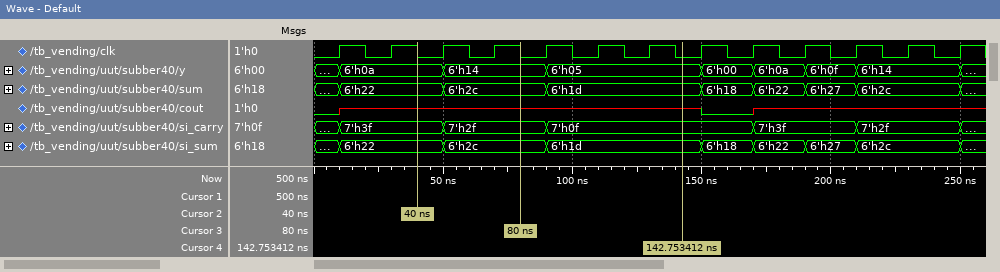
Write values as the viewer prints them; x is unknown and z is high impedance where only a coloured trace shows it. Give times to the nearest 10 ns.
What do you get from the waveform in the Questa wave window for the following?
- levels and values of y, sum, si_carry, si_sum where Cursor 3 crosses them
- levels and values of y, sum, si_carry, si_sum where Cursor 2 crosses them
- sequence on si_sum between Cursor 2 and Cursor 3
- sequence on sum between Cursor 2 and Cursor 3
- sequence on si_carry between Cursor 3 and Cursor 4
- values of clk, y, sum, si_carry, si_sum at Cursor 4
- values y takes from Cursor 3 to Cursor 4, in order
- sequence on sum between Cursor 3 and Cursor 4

y=6'h14, sum=6'h2c, si_carry=7'h2f, si_sum=6'h2c
y=6'h0a, sum=6'h22, si_carry=7'h3f, si_sum=6'h22
6'h22, 6'h2c
6'h22, 6'h2c
7'h2f, 7'h0f
clk=0, y=6'h05, sum=6'h1d, si_carry=7'h0f, si_sum=6'h1d
6'h14, 6'h05
6'h2c, 6'h1d
